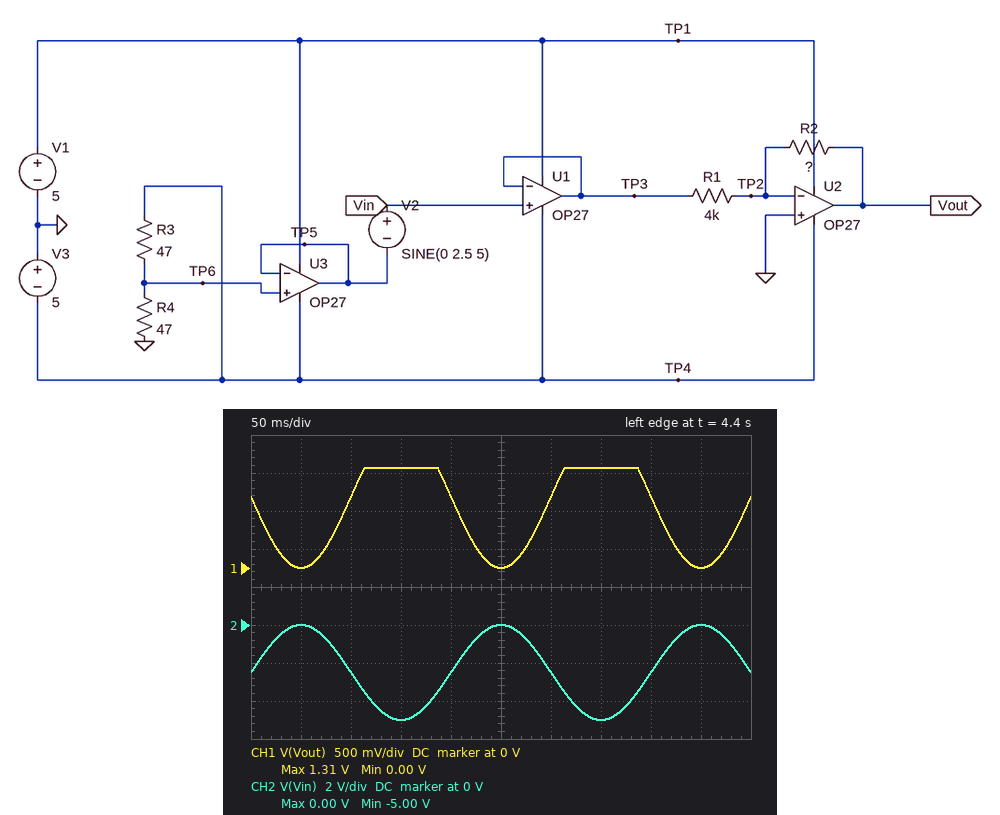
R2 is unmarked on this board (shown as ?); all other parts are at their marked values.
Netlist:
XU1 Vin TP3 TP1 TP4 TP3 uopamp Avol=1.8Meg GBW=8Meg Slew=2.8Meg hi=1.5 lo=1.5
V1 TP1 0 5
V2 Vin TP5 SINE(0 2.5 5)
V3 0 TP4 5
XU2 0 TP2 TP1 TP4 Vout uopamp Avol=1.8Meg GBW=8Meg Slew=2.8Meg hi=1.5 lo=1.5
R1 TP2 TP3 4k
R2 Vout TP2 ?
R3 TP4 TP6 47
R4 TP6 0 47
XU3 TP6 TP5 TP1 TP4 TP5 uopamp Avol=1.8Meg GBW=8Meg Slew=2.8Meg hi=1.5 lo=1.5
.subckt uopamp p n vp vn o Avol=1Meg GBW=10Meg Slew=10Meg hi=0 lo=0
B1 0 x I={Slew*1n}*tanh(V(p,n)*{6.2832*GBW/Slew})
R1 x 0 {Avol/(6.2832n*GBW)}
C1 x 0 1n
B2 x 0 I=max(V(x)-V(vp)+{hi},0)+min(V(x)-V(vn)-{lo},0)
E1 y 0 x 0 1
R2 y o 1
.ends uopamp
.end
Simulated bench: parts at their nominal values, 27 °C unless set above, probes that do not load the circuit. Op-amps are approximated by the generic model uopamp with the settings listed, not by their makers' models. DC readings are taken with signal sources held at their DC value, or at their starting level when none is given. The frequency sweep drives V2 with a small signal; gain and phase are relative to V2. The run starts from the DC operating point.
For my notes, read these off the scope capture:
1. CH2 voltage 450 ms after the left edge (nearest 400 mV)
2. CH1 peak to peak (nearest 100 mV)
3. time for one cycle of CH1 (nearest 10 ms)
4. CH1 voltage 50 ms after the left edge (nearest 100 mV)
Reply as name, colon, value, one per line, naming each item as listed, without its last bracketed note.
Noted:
CH2 voltage 450 ms after the left edge: 0 V
CH1 peak to peak: 1.3 V
time for one cycle of CH1: 200 ms
CH1 voltage 50 ms after the left edge: 0 V
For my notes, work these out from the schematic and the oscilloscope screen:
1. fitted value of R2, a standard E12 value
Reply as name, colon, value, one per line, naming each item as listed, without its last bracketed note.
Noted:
fitted value of R2, a standard E12 value: 1.5 kΩ
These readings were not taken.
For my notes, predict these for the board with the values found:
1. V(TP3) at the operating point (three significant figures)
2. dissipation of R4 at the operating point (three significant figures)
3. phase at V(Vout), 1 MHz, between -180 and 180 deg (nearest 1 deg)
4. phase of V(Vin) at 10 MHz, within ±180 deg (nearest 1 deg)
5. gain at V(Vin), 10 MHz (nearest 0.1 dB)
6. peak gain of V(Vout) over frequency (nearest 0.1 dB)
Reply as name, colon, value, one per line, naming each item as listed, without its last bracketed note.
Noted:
V(TP3) at the operating point: -2.50 V
dissipation of R4 at the operating point: 133 mW
phase at V(Vout), 1 MHz, between -180 and 180 deg: 163 deg
phase of V(Vin) at 10 MHz, within ±180 deg: 0 deg
gain at V(Vin), 10 MHz: 0 dB
peak gain of V(Vout) over frequency: -8.5 dB
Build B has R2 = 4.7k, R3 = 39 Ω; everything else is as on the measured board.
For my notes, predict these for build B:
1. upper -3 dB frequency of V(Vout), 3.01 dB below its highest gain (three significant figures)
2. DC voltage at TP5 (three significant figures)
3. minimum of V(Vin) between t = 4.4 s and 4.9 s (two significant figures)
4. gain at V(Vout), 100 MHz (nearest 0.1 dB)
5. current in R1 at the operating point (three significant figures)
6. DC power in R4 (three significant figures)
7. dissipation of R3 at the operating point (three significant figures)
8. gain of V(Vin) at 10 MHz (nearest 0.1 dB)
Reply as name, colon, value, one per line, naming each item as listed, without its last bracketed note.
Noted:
upper -3 dB frequency of V(Vout), 3.01 dB below its highest gain: 3.15 MHz
DC voltage at TP5: -2.73 V
minimum of V(Vin) between t = 4.4 s and 4.9 s: -5.2 V
gain at V(Vout), 100 MHz: -49.3 dB
current in R1 at the operating point: 683 µA
DC power in R4: 159 mW
dissipation of R3 at the operating point: 132 mW
gain of V(Vin) at 10 MHz: 0 dB
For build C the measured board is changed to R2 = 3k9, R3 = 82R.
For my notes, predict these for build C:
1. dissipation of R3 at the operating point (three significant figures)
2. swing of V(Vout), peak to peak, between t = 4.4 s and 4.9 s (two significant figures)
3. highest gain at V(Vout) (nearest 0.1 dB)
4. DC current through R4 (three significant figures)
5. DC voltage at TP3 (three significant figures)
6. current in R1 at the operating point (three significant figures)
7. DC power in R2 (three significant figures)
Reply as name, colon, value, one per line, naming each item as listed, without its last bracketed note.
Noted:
dissipation of R3 at the operating point: 123 mW
swing of V(Vout), peak to peak, between t = 4.4 s and 4.9 s: 4.1 V
highest gain at V(Vout): -0.2 dB
DC current through R4: 38.8 mA
DC voltage at TP3: -1.82 V
current in R1 at the operating point: 455 µA
DC power in R2: 809 µW
